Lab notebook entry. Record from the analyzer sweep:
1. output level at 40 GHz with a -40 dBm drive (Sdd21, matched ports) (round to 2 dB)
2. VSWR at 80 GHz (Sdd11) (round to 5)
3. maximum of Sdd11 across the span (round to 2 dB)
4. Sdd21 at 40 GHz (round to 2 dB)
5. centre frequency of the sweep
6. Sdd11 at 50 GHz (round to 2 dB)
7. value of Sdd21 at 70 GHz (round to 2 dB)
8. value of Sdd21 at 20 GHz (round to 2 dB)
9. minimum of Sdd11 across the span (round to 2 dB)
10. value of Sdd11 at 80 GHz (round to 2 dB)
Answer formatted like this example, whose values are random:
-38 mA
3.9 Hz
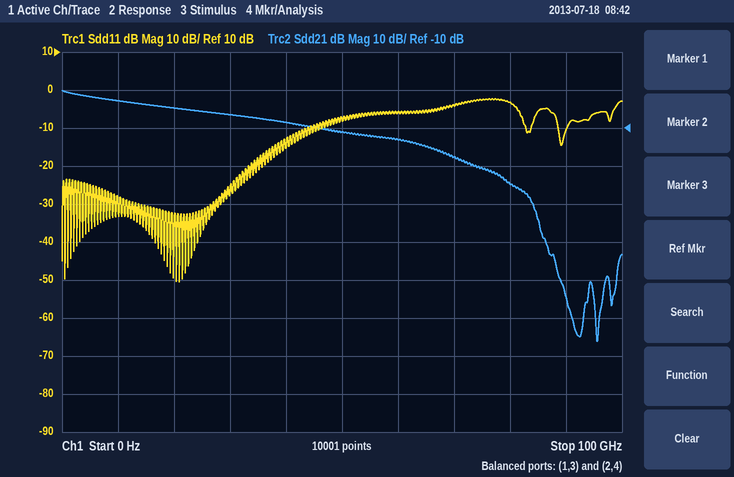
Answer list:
-48 dBm
5
-2 dB
-8 dB
50 GHz
-8 dB
-18 dB
-4 dB
-50 dB
-4 dB
